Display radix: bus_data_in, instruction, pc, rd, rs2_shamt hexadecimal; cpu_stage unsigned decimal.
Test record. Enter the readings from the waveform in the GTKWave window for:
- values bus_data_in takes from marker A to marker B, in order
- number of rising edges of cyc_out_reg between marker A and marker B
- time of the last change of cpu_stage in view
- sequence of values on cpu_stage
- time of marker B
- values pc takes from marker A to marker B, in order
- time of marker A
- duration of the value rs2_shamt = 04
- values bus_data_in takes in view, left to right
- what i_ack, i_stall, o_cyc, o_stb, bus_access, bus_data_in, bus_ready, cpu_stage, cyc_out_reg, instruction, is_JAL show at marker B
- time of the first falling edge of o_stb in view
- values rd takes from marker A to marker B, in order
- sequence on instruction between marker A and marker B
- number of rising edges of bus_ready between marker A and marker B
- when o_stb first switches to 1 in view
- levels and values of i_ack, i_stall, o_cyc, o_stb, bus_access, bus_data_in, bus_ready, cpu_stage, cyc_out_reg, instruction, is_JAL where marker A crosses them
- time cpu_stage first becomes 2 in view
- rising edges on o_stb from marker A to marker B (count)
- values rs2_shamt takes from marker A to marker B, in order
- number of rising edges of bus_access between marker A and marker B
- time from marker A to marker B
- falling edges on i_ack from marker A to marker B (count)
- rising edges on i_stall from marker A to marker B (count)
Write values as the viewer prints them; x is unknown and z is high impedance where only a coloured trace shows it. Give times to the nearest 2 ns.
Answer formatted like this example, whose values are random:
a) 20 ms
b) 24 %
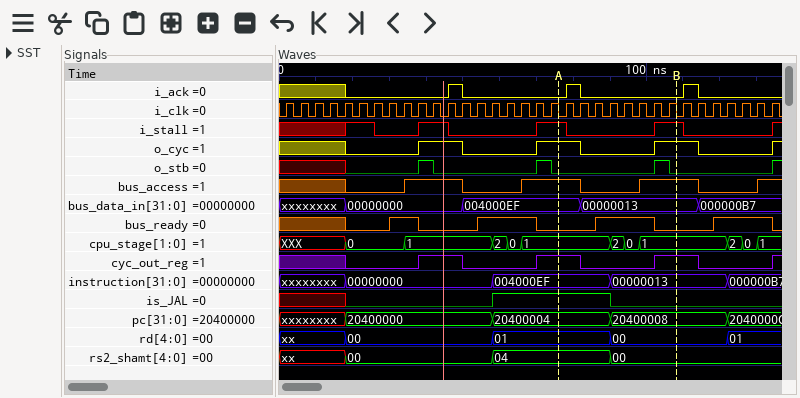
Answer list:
a) 004000EF, 00000013
b) 1
c) 130 ns
d) XXX, 0, 1, 2, 0, 1, 2, 0, 1, 2, 0, 1
e) 108 ns
f) 20400004, 20400008
g) 76 ns
h) 32 ns
i) xxxxxxxx, 00000000, 004000EF, 00000013, 000000B7
j) i_ack=0, i_stall=1, o_cyc=1, o_stb=0, bus_access=1, bus_data_in=00000013, bus_ready=0, cpu_stage=1, cyc_out_reg=1, instruction=00000013, is_JAL=0
k) 42 ns
l) 01, 00
m) 004000EF, 00000013
n) 1
o) 38 ns
p) i_ack=0, i_stall=1, o_cyc=1, o_stb=0, bus_access=1, bus_data_in=004000EF, bus_ready=0, cpu_stage=1, cyc_out_reg=1, instruction=004000EF, is_JAL=1
q) 58 ns
r) 1
s) 04, 00
t) 1
u) 32 ns
v) 1
w) 1
